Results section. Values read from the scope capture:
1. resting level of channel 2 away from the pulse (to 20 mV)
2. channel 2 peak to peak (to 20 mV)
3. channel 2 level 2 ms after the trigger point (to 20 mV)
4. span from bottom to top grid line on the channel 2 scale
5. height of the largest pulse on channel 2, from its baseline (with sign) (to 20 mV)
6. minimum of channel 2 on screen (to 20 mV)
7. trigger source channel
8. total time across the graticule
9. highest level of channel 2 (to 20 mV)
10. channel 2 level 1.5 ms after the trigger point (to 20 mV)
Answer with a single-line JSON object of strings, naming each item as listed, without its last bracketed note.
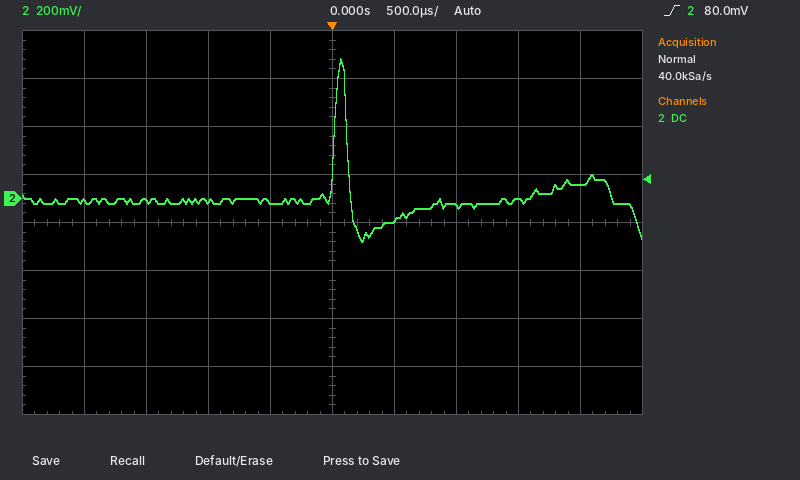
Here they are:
{"resting level of channel 2 away from the pulse": "-20 mV", "channel 2 peak to peak": "760 mV", "channel 2 level 2 ms after the trigger point": "60 mV", "span from bottom to top grid line on the channel 2 scale": "1.6 V", "height of the largest pulse on channel 2, from its baseline (with sign)": "+600 mV", "minimum of channel 2 on screen": "-180 mV", "trigger source channel": "channel 2", "total time across the graticule": "5 ms", "highest level of channel 2": "580 mV", "channel 2 level 1.5 ms after the trigger point": "0 mV"}
